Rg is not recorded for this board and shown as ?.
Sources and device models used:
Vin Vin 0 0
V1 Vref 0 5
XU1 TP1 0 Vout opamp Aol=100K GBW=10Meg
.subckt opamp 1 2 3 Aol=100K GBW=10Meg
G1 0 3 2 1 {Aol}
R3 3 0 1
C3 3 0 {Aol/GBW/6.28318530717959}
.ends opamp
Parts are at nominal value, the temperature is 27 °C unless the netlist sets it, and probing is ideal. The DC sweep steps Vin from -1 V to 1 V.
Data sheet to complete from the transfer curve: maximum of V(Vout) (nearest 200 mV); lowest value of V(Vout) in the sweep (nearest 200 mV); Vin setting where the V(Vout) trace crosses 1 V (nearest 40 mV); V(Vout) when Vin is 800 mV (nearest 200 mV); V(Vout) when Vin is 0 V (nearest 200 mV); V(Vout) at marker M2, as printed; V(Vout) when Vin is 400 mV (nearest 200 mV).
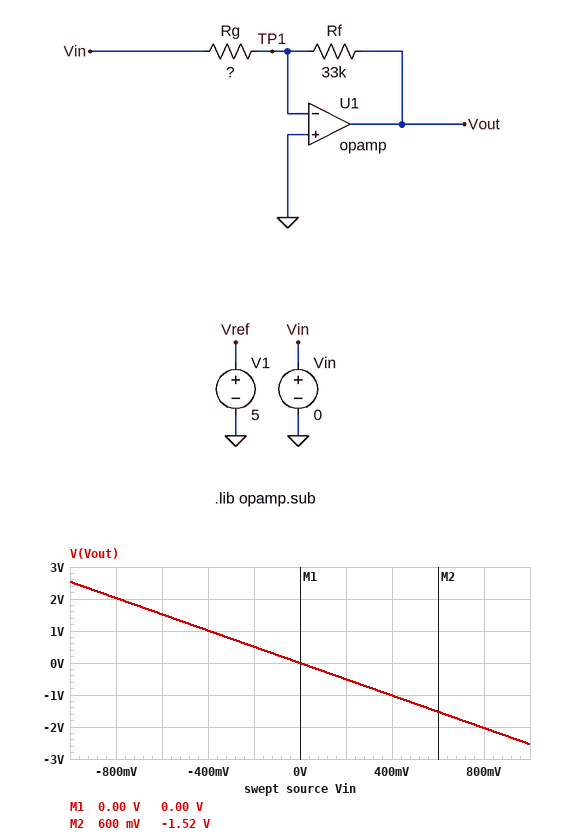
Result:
2.6 V
-2.6 V
-400 mV
-2.0 V
0 V
-1.52 V
-1.0 V
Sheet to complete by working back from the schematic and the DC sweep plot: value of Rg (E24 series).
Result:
13 kΩ
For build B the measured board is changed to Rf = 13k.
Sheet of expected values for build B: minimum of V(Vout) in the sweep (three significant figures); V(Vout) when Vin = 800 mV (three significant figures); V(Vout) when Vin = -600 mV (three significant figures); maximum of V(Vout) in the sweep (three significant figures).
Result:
-1.00 V
-800 mV
600 mV
1.00 V
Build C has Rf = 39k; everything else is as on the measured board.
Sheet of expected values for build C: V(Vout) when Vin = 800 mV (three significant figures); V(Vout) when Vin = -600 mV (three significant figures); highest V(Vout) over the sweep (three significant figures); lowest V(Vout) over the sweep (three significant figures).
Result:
-2.40 V
1.80 V
3.00 V
-3.00 V
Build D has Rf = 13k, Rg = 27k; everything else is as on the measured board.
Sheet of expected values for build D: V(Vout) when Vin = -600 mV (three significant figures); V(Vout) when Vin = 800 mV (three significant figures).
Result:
289 mV
-385 mV
